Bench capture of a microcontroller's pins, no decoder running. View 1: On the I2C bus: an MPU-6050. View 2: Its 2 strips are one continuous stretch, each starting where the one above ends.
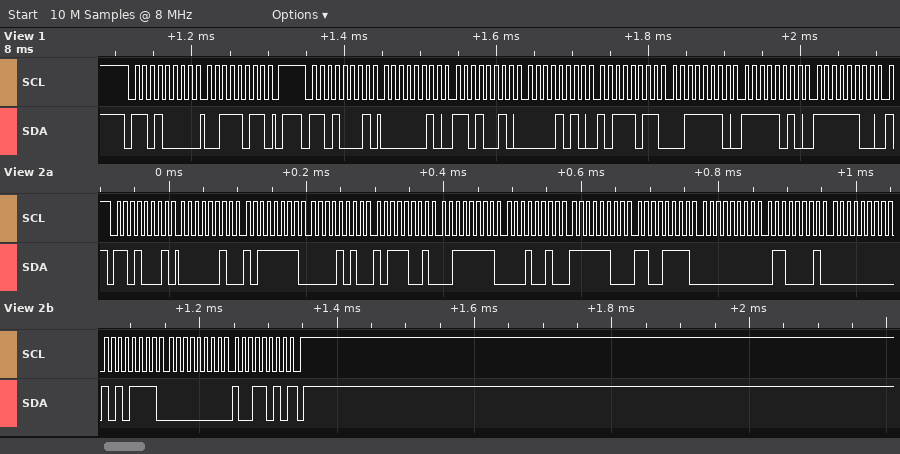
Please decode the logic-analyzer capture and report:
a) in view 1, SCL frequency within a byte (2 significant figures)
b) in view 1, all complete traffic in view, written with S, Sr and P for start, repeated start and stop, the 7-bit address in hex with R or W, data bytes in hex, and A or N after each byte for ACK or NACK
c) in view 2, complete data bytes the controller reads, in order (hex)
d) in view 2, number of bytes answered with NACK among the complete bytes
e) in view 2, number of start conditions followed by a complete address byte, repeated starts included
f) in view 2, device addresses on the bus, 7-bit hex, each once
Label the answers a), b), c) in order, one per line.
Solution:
a) 100 kHz
b) S 68W A 3B A P S 68R A 02 A D2 A 0A A BB A 3E A FA A FC A
c) 02 BF 0A B9 3F 12 FC CF 00 61 00 AF 00 9A
d) 1
e) 1
f) 0x68
